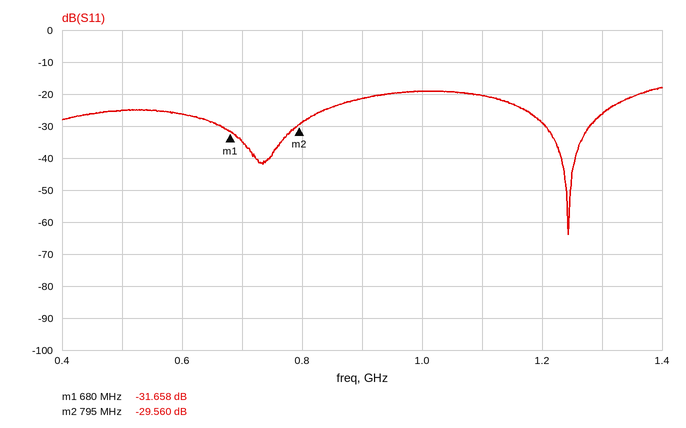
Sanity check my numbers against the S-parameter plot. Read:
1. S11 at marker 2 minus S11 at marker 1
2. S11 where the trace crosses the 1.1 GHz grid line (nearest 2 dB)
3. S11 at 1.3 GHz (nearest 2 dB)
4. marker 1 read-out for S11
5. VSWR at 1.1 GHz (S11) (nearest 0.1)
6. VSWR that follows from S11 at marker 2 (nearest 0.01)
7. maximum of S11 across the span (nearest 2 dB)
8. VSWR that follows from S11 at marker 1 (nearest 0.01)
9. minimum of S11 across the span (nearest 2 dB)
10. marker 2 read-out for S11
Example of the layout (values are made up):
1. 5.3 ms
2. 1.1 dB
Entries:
1. 2.098 dB
2. -20 dB
3. -26 dB
4. -31.658 dB
5. 1.2
6. 1.07
7. -18 dB
8. 1.05
9. -64 dB
10. -29.560 dB
